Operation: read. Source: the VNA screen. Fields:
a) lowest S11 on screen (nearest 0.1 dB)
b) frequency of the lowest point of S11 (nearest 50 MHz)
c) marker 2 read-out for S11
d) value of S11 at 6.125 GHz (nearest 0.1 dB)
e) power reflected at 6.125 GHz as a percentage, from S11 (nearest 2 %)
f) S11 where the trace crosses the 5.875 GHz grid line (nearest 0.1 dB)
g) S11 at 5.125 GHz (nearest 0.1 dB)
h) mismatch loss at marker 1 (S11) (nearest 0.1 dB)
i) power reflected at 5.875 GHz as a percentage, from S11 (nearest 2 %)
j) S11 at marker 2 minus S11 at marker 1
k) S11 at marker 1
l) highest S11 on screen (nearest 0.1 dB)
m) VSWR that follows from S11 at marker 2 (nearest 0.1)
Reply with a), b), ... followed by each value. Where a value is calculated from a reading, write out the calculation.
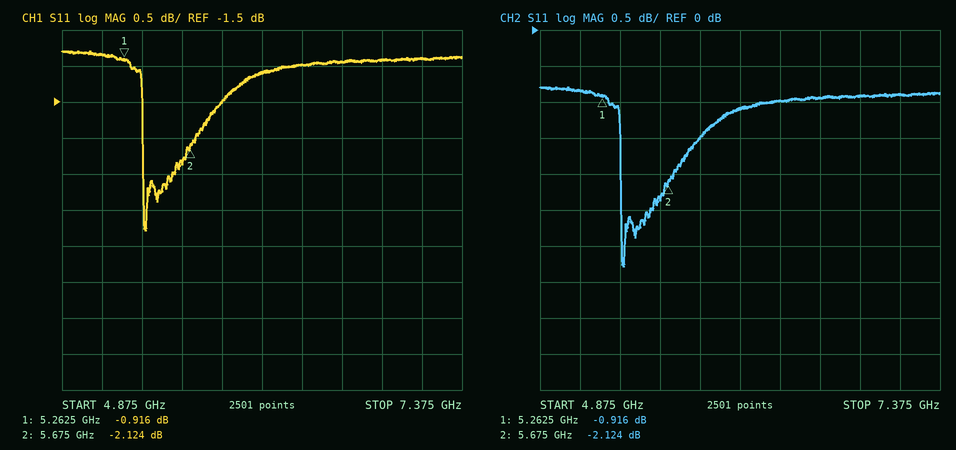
a) -3.3 dB
b) 5.40 GHz
c) -2.124 dB
d) -1.1 dB
e) 10^(-1.1/10) ≈ 78 %
f) -1.5 dB
g) -0.8 dB
h) −10 log10(1 − 10^(-0.916/10)) ≈ 7.2 dB
i) 10^(-1.5/10) ≈ 70.8 %, so 70 % to the nearest 2 %
j) -2.124 − (-0.916) = -1.208 dB
k) -0.916 dB
l) -0.8 dB
m) (1 + 0.7831)/(1 − 0.7831) ≈ 8.2
